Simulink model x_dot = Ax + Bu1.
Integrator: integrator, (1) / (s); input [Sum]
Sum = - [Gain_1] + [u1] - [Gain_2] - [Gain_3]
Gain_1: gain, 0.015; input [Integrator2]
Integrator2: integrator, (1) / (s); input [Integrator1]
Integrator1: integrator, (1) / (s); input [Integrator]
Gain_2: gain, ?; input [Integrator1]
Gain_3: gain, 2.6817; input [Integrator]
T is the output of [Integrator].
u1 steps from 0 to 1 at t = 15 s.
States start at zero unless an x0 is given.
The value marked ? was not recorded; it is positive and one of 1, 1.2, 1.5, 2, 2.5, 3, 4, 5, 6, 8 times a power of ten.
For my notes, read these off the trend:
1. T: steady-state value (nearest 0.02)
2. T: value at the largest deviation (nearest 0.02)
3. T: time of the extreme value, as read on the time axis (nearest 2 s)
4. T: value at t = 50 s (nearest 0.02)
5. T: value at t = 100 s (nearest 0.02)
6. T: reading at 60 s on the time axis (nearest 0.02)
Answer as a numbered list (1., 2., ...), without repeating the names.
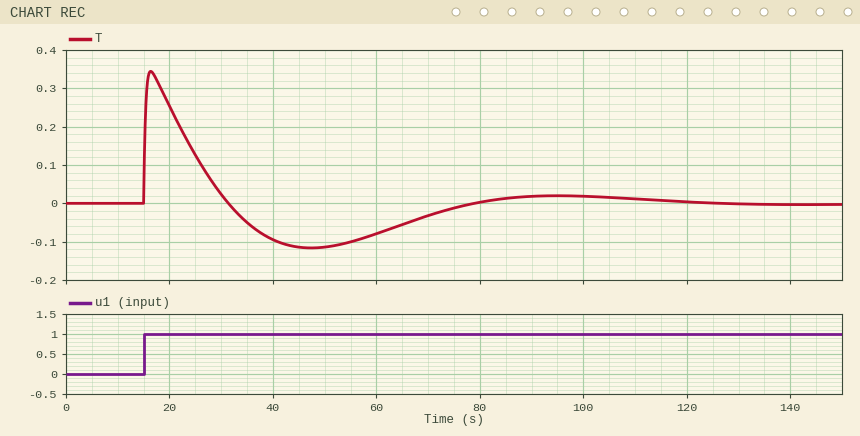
1. 0.00
2. 0.34
3. 16 s
4. -0.12
5. 0.02
6. -0.08
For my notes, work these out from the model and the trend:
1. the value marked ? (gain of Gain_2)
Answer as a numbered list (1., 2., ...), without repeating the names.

1. 0.2
